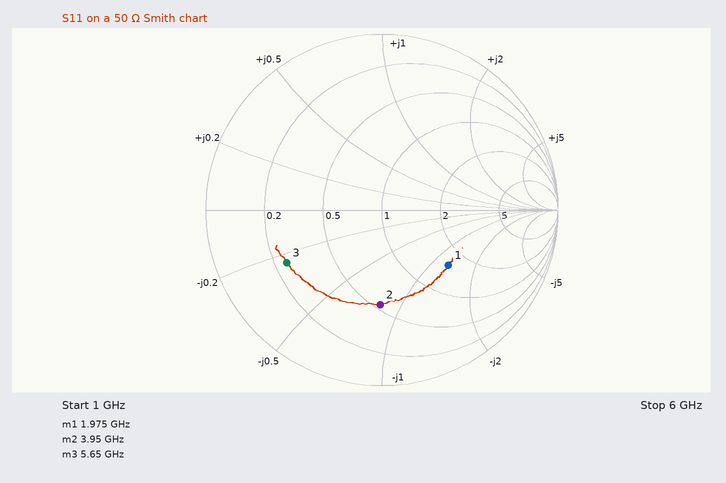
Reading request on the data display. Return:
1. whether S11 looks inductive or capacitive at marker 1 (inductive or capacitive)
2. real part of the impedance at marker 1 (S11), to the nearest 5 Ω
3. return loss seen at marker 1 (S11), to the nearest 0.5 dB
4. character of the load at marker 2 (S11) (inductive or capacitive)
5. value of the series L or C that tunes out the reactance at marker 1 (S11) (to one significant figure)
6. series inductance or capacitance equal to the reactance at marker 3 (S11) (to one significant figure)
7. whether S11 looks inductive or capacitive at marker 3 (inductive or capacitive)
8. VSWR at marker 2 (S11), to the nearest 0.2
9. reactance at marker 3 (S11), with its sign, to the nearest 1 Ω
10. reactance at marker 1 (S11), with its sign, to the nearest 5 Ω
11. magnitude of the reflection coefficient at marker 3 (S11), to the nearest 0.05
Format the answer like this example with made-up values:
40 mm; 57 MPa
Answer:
capacitive; 80 Ω; 6.0 dB; capacitive; 5 nH; 2 pF; capacitive; 3.4; -12 Ω; -65 Ω; 0.60
